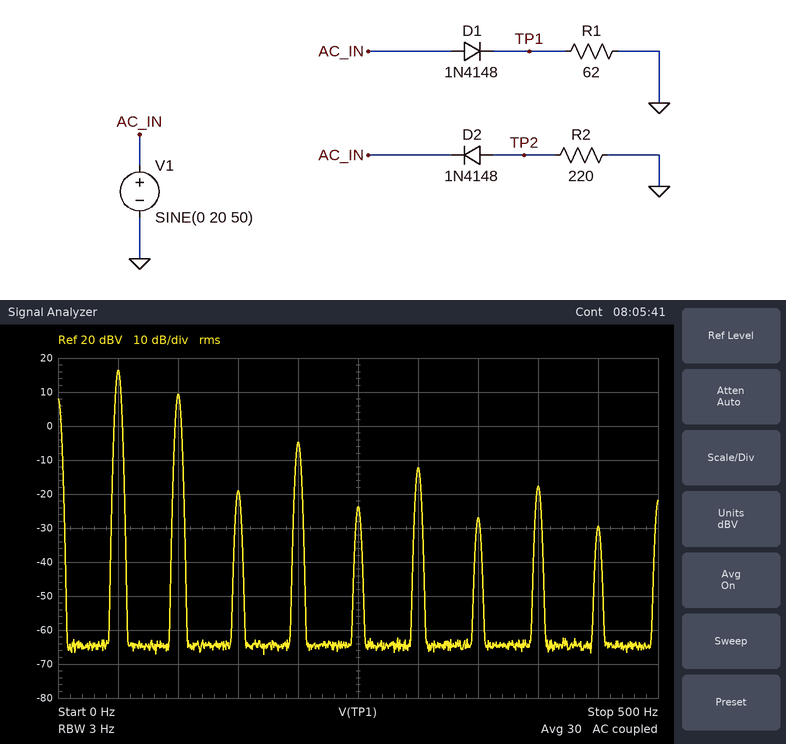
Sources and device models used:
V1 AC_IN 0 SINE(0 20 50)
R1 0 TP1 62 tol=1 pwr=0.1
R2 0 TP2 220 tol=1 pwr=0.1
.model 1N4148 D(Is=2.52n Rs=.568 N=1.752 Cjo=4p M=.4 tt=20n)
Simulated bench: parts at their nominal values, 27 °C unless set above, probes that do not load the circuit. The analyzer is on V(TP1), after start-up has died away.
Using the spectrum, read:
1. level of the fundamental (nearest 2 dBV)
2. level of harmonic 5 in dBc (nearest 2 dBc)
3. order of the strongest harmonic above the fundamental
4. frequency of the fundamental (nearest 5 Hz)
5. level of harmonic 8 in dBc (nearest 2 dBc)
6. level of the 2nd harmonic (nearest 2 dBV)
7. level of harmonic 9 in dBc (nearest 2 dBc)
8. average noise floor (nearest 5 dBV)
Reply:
16 dBV
-40 dBc
2
50 Hz
-34 dBc
10 dBV
-46 dBc
-65 dBV
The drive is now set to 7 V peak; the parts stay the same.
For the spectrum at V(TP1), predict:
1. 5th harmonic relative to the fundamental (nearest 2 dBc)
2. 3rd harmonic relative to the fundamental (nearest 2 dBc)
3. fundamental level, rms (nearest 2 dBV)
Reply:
-32 dBc
-26 dBc
6 dBV
